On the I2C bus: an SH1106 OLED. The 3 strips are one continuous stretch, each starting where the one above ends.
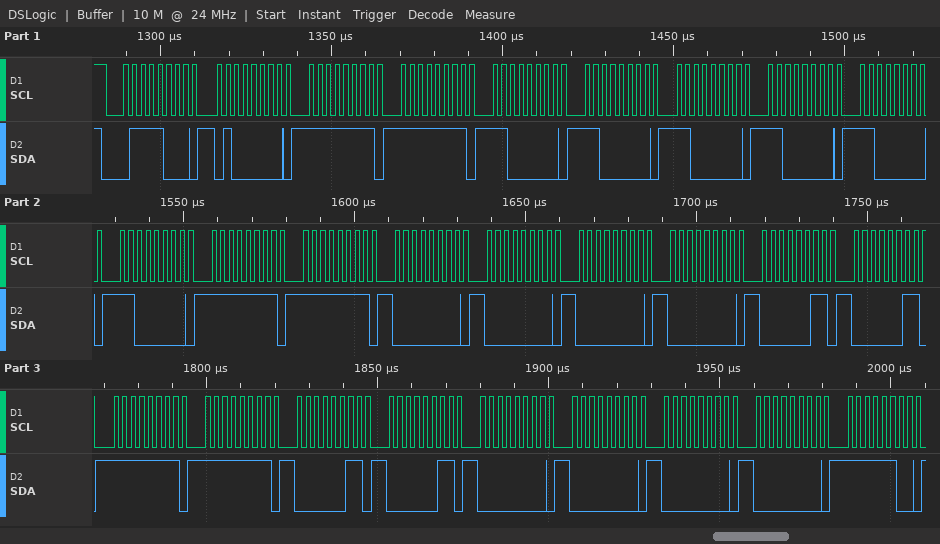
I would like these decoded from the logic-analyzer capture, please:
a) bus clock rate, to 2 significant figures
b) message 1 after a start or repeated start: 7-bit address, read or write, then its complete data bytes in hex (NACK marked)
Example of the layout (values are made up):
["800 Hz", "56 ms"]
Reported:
["400 kHz", "0x3C write: 40 FF FF C0 C0 C0 C0 C0 C0 FF FF 00 00 00 00 03 03 FF FF 03 03 00 00 00 00 FC"]
